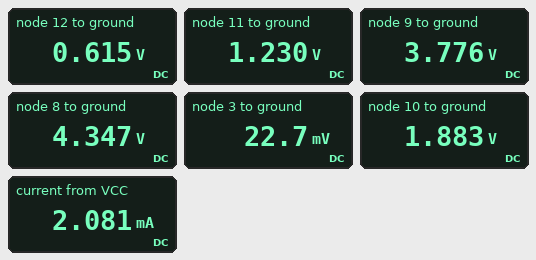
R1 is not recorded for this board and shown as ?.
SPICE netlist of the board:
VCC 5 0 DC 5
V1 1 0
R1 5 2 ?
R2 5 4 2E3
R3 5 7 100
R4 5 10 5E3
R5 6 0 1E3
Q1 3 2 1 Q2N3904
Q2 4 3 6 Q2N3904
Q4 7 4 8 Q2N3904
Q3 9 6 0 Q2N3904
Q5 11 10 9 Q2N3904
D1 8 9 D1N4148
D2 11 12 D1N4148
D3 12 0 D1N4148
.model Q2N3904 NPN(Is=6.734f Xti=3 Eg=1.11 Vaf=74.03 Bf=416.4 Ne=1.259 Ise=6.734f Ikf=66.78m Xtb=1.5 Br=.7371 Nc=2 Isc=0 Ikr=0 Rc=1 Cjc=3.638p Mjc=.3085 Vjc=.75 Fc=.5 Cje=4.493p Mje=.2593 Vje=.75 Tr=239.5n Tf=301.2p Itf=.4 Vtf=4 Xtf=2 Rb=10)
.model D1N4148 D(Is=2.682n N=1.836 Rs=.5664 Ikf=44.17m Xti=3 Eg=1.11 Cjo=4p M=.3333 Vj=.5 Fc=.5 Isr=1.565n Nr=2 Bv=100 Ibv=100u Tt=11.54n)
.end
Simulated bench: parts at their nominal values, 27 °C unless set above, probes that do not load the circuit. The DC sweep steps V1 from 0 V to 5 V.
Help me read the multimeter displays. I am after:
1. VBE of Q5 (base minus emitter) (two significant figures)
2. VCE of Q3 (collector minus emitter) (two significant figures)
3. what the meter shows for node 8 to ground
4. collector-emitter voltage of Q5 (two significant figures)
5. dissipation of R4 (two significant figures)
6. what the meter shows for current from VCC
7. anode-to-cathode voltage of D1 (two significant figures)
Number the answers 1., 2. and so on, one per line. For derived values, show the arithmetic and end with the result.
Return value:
1. 1.883 V - 3.776 V = -1.9 V
2. 3.776 V = 3.8 V
3. 4.347 V
4. 1.23 V - 3.776 V = -2.5 V
5. (5 V - 1.883 V)^2 / 5 kΩ = 1.9 mW
6. 2.081 mA
7. 4.347 V - 3.776 V = 570 mV
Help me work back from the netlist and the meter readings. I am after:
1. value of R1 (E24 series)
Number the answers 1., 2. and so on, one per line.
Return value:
1. 4.3 kΩ
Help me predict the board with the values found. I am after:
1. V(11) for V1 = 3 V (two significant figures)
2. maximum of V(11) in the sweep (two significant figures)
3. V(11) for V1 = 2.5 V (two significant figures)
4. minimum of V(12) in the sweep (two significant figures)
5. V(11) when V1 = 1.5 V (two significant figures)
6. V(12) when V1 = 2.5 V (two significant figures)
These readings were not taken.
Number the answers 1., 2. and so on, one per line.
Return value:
1. 52 mV
2. 1.2 V
3. 52 mV
4. 26 mV
5. 52 mV
6. 26 mV
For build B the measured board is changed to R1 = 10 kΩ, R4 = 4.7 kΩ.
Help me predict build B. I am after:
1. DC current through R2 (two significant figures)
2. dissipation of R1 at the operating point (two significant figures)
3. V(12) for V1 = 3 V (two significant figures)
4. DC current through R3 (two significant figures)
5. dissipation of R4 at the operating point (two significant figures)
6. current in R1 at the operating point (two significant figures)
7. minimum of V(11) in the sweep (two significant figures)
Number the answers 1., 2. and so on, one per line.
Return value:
1. 4.0 µA
2. 1.9 mW
3. 27 mV
4. 480 µA
5. 2.1 mW
6. 430 µA
7. 53 mV
